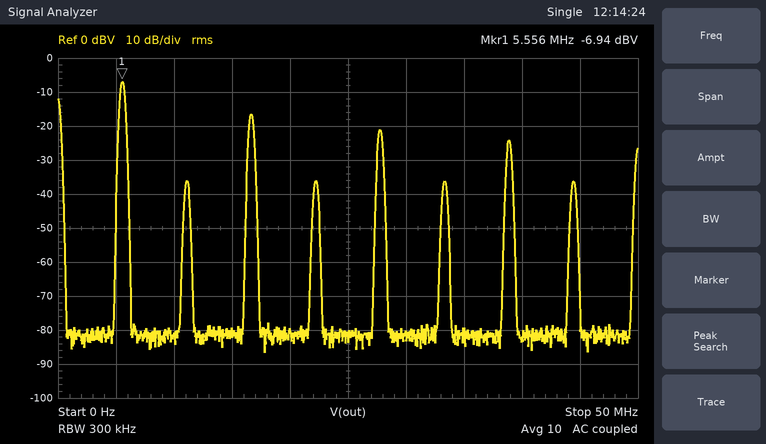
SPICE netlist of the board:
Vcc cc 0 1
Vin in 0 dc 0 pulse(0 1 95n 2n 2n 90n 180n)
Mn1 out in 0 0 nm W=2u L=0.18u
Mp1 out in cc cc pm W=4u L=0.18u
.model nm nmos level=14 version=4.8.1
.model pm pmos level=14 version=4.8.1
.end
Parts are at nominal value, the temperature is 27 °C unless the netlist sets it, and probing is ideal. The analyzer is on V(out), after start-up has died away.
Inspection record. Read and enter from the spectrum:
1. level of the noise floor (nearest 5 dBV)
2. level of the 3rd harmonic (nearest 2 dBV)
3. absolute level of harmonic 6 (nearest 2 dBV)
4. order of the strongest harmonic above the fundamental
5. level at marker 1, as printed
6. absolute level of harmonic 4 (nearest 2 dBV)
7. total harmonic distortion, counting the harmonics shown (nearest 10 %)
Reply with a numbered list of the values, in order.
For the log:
1. -80 dBV
2. -16 dBV
3. -36 dBV
4. 3
5. -6.94 dBV
6. -36 dBV
7. 40 %
